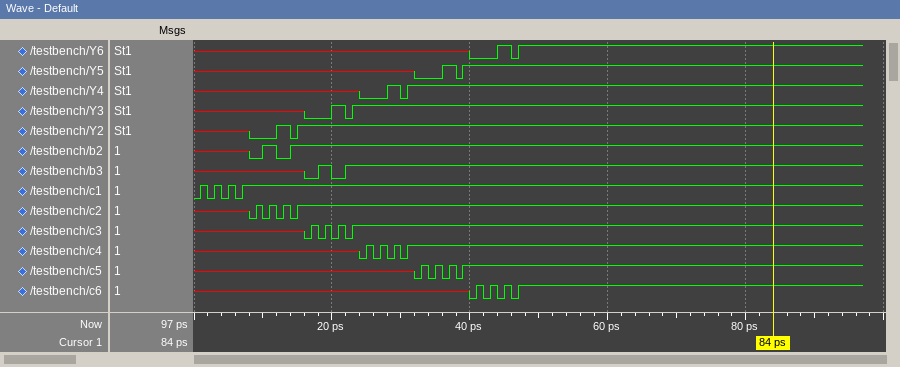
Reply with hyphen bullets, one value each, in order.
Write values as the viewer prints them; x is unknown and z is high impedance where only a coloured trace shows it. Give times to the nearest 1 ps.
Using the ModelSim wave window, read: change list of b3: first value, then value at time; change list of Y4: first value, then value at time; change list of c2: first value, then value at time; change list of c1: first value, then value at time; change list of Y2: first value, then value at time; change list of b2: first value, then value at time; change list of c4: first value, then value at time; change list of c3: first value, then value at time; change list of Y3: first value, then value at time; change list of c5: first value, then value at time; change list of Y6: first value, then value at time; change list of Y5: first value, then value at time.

- x, 0 at 16 ps, 1 at 18 ps, 0 at 20 ps, 1 at 22 ps
- x, 0 at 24 ps, 1 at 28 ps, 0 at 30 ps, 1 at 31 ps
- x, 0 at 8 ps, 1 at 9 ps, 0 at 10 ps, 1 at 11 ps, 0 at 12 ps, 1 at 13 ps, 0 at 14 ps, 1 at 15 ps
- 0, 1 at 1 ps, 0 at 2 ps, 1 at 3 ps, 0 at 4 ps, 1 at 5 ps, 0 at 6 ps, 1 at 7 ps
- x, 0 at 8 ps, 1 at 12 ps, 0 at 14 ps, 1 at 15 ps
- x, 0 at 8 ps, 1 at 10 ps, 0 at 12 ps, 1 at 14 ps
- x, 0 at 24 ps, 1 at 25 ps, 0 at 26 ps, 1 at 27 ps, 0 at 28 ps, 1 at 29 ps, 0 at 30 ps, 1 at 31 ps
- x, 0 at 16 ps, 1 at 17 ps, 0 at 18 ps, 1 at 19 ps, 0 at 20 ps, 1 at 21 ps, 0 at 22 ps, 1 at 23 ps
- x, 0 at 16 ps, 1 at 20 ps, 0 at 22 ps, 1 at 23 ps
- x, 0 at 32 ps, 1 at 33 ps, 0 at 34 ps, 1 at 35 ps, 0 at 36 ps, 1 at 37 ps, 0 at 38 ps, 1 at 39 ps
- x, 0 at 40 ps, 1 at 44 ps, 0 at 46 ps, 1 at 47 ps
- x, 0 at 32 ps, 1 at 36 ps, 0 at 38 ps, 1 at 39 ps
